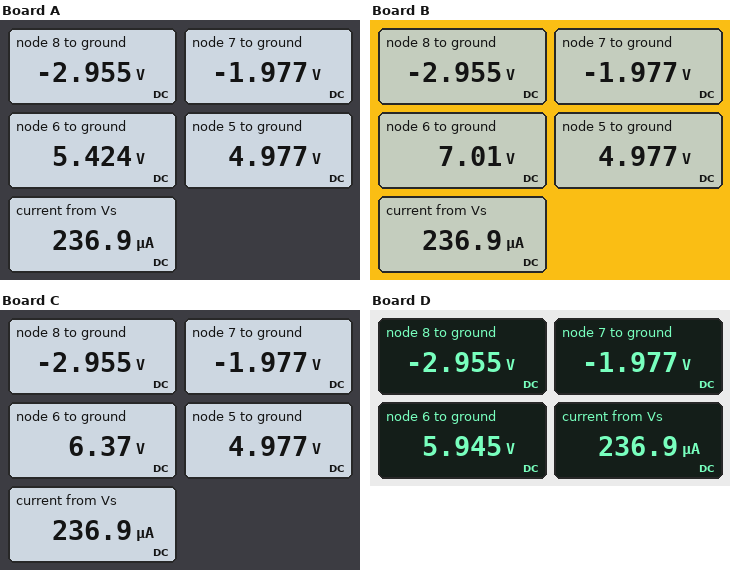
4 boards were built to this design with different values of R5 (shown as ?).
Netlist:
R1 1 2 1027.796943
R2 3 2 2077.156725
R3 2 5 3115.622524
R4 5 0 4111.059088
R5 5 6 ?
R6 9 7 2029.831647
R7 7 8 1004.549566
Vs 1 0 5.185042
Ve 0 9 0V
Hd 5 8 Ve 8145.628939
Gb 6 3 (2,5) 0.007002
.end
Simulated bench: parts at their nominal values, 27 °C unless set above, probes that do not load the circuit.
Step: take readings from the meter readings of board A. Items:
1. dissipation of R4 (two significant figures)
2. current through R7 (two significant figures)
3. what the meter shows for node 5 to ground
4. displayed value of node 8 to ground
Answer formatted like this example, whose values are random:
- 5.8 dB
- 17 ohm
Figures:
- 6.0 mW
- 970 µA
- 4.977 V
- -2.955 V
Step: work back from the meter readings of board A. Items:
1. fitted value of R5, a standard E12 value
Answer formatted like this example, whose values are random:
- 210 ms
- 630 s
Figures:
- 1.8 kΩ
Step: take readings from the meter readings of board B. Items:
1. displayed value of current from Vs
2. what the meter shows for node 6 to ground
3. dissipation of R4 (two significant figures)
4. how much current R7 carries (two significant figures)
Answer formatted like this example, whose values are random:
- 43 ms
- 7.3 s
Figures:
- 236.9 µA
- 7.01 V
- 6.0 mW
- 970 µA
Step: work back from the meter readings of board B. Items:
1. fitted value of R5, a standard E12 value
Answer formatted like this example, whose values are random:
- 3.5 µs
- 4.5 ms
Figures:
- 8.2 kΩ
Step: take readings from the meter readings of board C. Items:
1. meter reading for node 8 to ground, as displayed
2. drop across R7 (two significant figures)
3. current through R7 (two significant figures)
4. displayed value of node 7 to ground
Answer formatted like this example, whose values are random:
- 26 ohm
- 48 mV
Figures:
- -2.955 V
- 980 mV
- 970 µA
- -1.977 V
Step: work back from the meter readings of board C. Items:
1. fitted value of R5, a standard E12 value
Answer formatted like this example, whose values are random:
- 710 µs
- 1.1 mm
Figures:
- 5.6 kΩ
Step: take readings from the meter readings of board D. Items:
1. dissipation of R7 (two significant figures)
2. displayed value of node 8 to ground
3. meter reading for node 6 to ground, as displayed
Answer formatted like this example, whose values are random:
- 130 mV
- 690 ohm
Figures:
- 950 µW
- -2.955 V
- 5.945 V
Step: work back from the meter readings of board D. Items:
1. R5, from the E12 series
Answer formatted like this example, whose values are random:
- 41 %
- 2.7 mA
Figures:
- 3.9 kΩ
